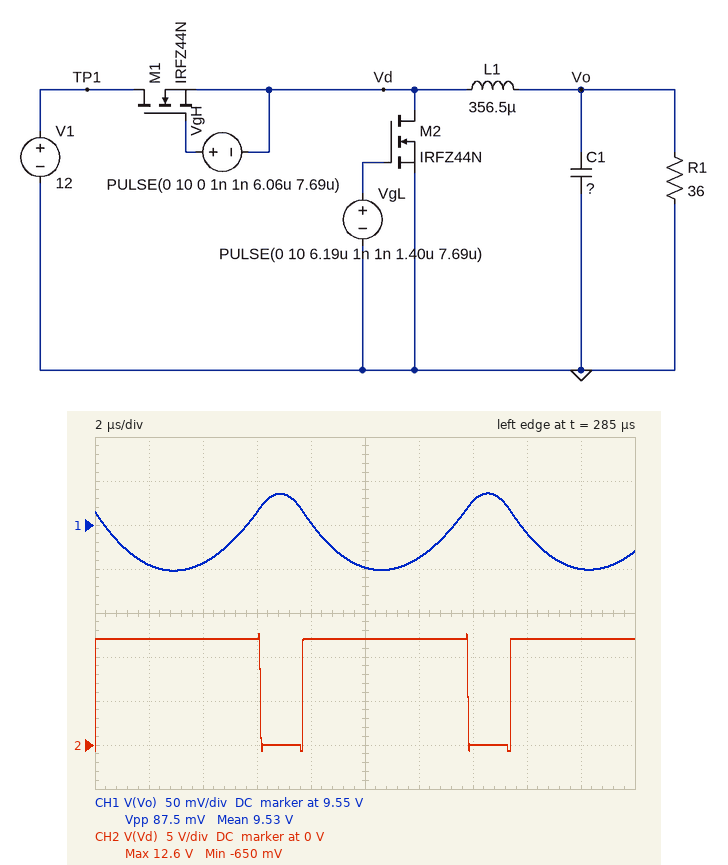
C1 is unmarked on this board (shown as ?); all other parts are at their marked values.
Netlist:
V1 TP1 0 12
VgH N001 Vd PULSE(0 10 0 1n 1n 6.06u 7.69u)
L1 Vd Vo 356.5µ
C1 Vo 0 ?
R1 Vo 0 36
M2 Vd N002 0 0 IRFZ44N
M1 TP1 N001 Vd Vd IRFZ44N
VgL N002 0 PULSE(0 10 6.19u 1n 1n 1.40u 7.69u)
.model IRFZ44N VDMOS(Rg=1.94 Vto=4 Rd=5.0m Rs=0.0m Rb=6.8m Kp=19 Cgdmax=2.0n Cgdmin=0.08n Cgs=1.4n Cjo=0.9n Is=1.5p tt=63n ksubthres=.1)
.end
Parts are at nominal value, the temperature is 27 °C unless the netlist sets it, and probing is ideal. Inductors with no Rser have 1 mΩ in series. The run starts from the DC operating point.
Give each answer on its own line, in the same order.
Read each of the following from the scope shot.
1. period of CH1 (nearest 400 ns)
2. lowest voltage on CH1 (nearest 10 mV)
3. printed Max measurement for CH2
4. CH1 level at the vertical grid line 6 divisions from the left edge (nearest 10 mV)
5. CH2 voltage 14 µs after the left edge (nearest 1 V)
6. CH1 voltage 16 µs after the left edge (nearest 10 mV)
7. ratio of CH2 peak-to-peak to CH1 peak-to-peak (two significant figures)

7.6 µs
9.50 V
12.6 V
9.51 V
0 V
9.54 V
150
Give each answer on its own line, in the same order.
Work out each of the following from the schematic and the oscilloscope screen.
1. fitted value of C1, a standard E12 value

470 nF
